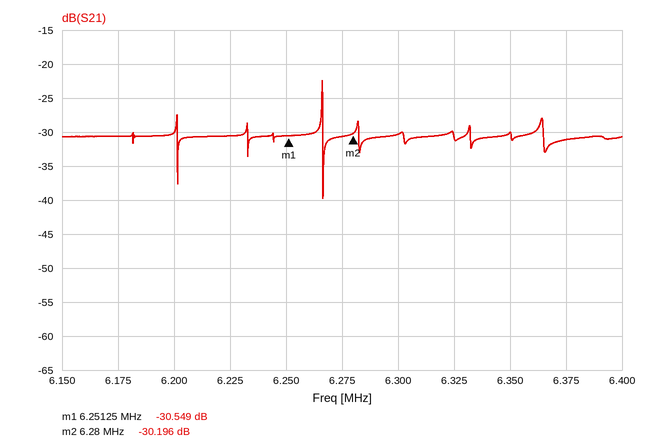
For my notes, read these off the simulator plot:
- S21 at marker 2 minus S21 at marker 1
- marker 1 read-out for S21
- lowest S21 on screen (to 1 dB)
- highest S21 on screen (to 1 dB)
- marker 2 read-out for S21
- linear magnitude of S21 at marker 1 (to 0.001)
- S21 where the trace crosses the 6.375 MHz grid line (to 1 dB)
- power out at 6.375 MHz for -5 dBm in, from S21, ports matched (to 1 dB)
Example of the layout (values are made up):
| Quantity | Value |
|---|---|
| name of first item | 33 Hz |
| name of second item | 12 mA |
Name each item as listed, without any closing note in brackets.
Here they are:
| Quantity | Value |
|---|---|
| S21 at marker 2 minus S21 at marker 1 | 0.353 dB |
| marker 1 read-out for S21 | -30.549 dB |
| lowest S21 on screen | -40 dB |
| highest S21 on screen | -22 dB |
| marker 2 read-out for S21 | -30.196 dB |
| linear magnitude of S21 at marker 1 | 0.030 |
| S21 where the trace crosses the 6.375 MHz grid line | -31 dB |
| power out at 6.375 MHz for -5 dBm in, from S21, ports matched | -36 dBm |
